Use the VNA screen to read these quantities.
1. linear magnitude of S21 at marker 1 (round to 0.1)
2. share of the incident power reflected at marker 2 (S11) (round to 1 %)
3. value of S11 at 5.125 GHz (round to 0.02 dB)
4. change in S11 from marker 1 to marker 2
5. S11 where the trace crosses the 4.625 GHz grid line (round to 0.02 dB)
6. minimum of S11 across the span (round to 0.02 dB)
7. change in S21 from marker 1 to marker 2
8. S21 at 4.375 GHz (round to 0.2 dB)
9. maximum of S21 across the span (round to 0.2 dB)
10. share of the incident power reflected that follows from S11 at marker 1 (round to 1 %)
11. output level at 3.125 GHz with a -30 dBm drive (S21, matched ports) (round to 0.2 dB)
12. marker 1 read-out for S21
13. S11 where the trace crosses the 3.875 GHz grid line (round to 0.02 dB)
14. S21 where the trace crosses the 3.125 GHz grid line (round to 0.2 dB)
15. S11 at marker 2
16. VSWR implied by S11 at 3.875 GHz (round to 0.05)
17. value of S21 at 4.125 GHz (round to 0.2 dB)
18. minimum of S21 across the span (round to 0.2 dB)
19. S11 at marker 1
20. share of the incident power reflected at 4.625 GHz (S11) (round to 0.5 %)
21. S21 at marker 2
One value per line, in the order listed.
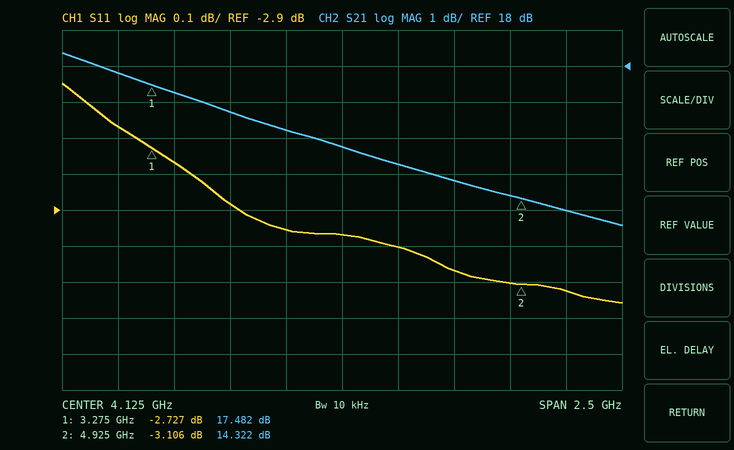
7.5
49 %
-3.12 dB
-0.379 dB
-3.06 dB
-3.16 dB
-3.160 dB
15.2 dB
18.4 dB
53 %
-12.2 dBm
17.482 dB
-2.96 dB
17.8 dB
-3.106 dB
5.95
15.8 dB
13.6 dB
-2.727 dB
49.5 %
14.322 dB
